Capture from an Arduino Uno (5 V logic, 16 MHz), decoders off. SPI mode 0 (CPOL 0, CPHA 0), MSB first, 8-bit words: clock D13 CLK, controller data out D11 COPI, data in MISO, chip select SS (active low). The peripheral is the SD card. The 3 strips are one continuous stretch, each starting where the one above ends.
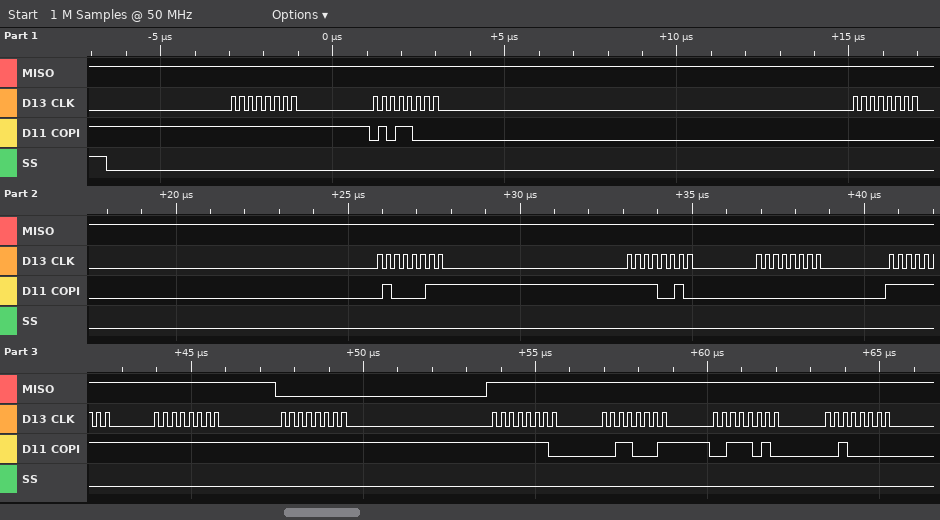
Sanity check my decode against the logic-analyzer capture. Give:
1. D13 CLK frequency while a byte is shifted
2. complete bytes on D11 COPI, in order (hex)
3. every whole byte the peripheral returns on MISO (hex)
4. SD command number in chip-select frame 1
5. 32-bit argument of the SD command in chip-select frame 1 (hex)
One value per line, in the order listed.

4 MHz
FF 58 00 43 F2 00 FF FF FF FE 31 3A 20
FF FF FF FF FF FF FF FF 00 FF FF FF FF
CMD24
0x0043F200
